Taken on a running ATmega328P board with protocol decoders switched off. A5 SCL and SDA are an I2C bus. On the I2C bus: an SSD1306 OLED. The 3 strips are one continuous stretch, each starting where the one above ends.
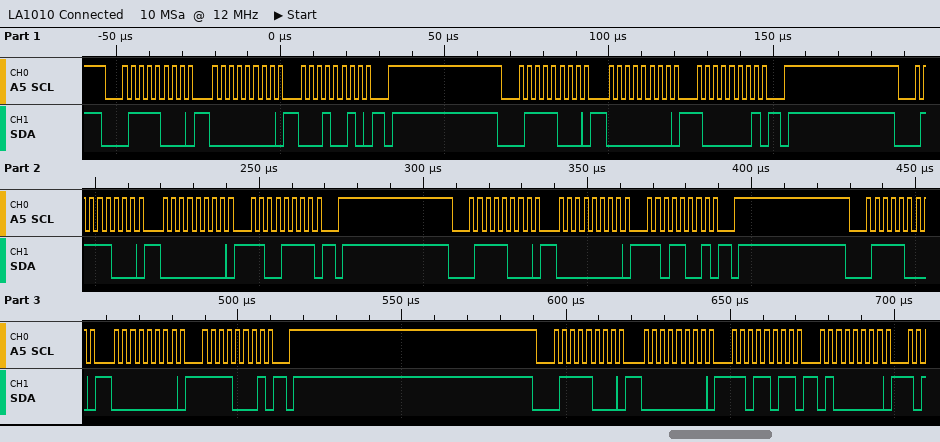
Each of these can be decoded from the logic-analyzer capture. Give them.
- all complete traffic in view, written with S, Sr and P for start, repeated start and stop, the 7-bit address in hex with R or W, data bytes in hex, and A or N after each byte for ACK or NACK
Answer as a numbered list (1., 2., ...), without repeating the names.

1. S 3CW A 00 A 12 A P S 3CW A 00 A 81 A P S 3CW A 00 A CF A P S 3CW A 00 A D9 A P S 3CW A 00 A F1 A P S 3CW A 00 A DB A 40 A
